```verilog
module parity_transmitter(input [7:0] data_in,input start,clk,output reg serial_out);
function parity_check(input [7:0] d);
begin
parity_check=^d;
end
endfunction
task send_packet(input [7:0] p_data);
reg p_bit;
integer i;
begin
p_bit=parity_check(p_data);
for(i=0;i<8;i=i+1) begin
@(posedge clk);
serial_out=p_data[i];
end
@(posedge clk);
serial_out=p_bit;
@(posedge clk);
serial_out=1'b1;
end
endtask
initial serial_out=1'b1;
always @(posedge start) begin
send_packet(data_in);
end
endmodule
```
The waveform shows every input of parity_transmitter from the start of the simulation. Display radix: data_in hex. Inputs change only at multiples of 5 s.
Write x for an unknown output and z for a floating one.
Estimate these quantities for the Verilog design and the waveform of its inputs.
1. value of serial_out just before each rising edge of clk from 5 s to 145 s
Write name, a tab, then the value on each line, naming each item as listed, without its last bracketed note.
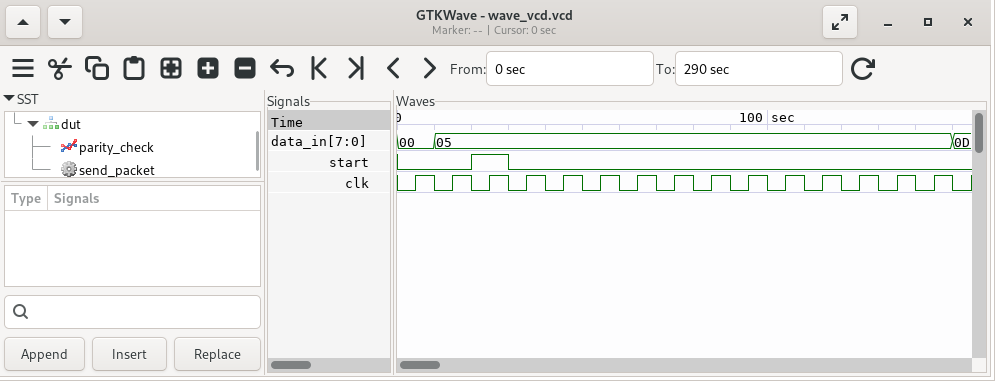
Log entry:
value of serial_out just before each rising edge of clk from 5 s to 145 s	1 1 1 1 0 1 0 0 0 0 0 0 1 1 1
